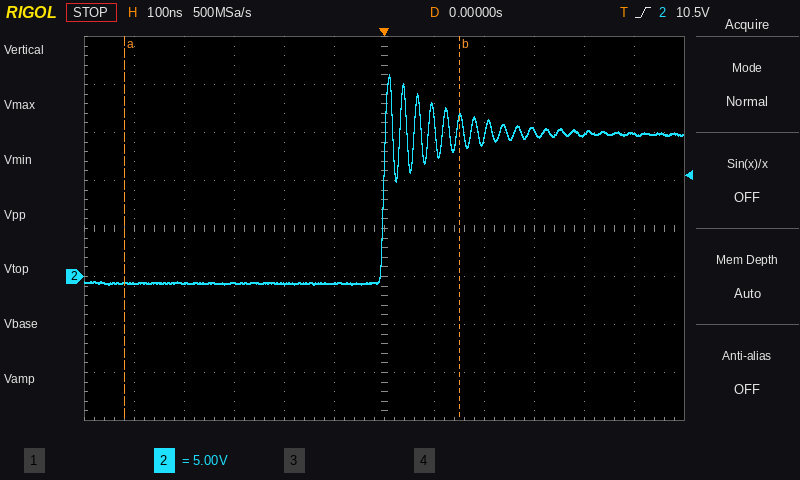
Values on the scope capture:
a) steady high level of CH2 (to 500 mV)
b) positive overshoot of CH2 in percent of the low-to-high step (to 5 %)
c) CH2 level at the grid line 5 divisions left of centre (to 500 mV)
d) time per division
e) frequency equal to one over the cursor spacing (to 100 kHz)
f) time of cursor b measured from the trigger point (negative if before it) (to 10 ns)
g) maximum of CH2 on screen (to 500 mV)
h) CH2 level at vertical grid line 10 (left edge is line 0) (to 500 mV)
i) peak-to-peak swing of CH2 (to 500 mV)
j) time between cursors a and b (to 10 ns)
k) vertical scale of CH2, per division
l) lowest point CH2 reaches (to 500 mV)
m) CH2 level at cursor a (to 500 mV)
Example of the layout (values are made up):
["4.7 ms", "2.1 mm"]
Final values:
["15.0 V", "40 %", "-500 mV", "100 ns", "1.5 MHz", "+150 ns", "21.0 V", "15.0 V", "22.0 V", "670 ns", "5 V", "-1.0 V", "-500 mV"]
